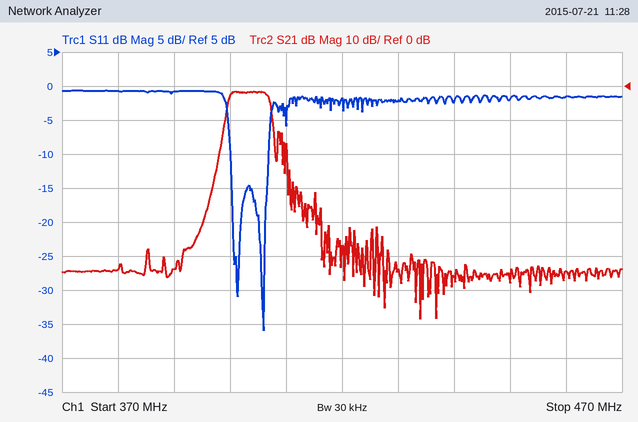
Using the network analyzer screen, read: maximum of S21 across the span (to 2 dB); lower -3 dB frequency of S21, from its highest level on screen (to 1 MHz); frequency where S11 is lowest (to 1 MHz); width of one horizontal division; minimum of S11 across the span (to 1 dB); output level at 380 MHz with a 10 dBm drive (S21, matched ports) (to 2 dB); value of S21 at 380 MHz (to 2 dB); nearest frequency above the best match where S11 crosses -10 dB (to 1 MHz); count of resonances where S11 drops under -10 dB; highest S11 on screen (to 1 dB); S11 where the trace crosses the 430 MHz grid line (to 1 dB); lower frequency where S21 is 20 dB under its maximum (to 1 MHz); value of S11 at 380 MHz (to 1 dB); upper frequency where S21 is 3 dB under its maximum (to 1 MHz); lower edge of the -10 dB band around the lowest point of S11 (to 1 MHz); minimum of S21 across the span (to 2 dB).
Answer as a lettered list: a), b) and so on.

a) -2 dB
b) 400 MHz
c) 406 MHz
d) 10 MHz
e) -36 dB
f) -44 dBm
g) -54 dB
h) 407 MHz
i) 2
j) -1 dB
k) -2 dB
l) 398 MHz
m) -1 dB
n) 407 MHz
o) 400 MHz
p) -68 dB
